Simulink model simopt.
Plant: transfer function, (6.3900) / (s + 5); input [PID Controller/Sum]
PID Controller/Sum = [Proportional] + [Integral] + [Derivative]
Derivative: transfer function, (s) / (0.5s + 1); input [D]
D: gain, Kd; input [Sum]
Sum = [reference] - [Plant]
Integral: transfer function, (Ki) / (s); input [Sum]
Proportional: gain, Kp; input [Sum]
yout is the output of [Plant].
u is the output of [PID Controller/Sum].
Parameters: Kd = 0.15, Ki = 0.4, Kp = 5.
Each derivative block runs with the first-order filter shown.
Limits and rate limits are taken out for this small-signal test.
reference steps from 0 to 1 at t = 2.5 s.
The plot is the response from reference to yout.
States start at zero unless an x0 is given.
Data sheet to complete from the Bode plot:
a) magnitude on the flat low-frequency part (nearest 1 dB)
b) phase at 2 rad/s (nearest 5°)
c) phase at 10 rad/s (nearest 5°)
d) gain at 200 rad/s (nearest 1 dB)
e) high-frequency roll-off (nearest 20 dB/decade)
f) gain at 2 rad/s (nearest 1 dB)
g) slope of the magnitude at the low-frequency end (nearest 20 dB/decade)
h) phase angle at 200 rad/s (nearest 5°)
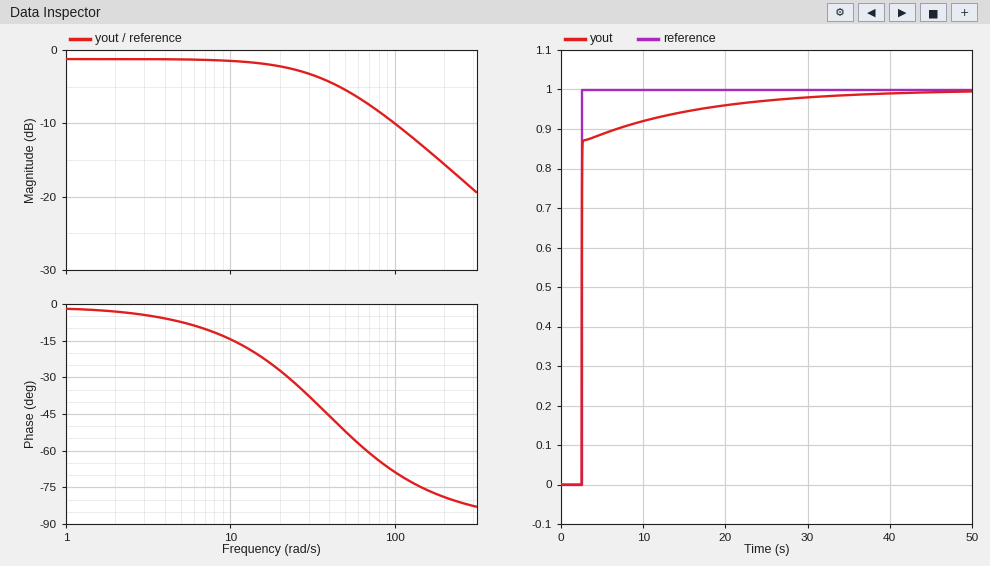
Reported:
-1 dB
-5°
-15°
-16 dB
-20 dB/decade
-1 dB
0 dB/decade
-80°
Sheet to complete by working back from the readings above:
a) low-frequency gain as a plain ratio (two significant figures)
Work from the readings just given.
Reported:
0.89
